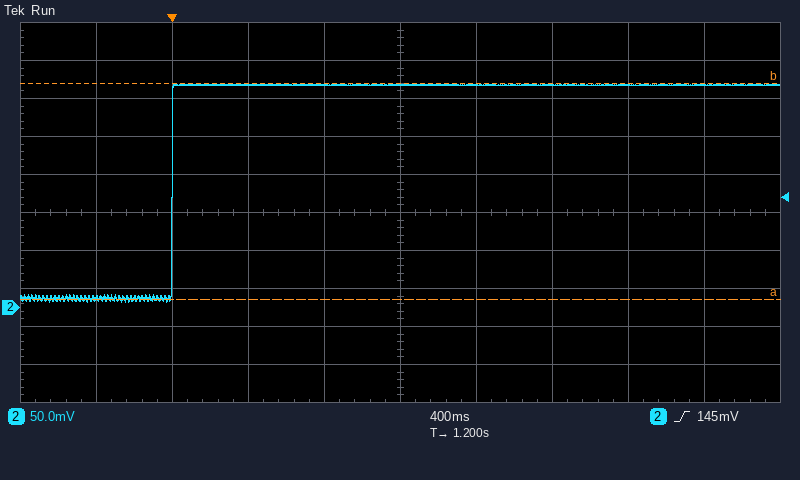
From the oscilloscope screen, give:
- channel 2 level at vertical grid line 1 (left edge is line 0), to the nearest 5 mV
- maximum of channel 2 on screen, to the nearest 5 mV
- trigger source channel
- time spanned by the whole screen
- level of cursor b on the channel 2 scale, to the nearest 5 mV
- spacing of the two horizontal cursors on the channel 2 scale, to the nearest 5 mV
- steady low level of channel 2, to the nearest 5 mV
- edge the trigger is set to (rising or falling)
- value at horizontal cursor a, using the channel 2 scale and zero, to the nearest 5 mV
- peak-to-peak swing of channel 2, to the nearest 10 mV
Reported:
10 mV
295 mV
channel 2
4 s
295 mV
285 mV
10 mV
rising
10 mV
290 mV
